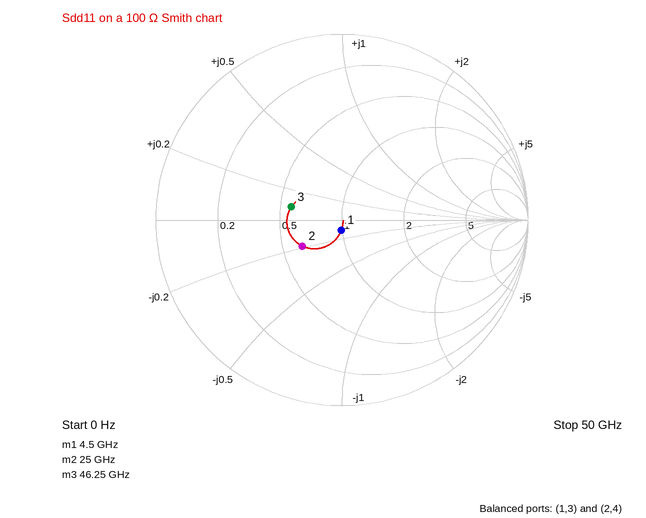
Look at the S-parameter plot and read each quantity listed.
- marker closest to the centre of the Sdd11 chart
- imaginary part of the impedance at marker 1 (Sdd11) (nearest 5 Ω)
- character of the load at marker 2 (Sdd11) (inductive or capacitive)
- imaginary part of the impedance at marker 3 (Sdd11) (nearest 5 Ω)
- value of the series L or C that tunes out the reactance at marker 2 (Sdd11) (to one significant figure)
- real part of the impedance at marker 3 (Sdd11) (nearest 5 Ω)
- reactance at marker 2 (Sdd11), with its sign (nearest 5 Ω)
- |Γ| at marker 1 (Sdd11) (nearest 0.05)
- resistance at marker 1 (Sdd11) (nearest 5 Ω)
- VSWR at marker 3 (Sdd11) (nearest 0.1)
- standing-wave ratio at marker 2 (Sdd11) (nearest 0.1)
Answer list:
marker 1
-10 Ω
capacitive
+10 Ω
100 pH
55 Ω
-20 Ω
0.05
100 Ω
1.8
1.7
